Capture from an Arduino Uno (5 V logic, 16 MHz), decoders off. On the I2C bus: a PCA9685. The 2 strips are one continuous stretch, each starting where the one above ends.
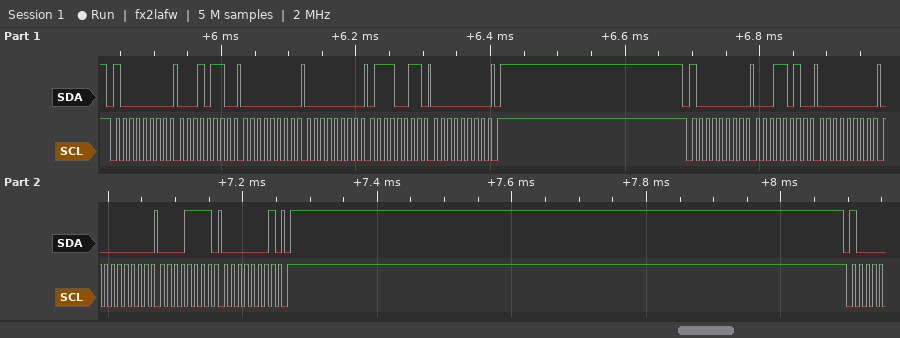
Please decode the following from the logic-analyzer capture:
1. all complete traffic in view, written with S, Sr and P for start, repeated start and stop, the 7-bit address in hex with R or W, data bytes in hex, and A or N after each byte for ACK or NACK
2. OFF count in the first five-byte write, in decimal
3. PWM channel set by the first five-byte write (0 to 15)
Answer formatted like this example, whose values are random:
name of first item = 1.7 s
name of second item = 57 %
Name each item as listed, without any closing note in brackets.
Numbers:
all complete traffic in view, written with S, Sr and P for start, repeated start and stop, the 7-bit address in hex with R or W, data bytes in hex, and A or N after each byte for ACK or NACK = S 40W A 16 A 00 A 00 A 73 A 00 A P S 40W A 1A A 00 A 00 A 0F A 01 A P
OFF count in the first five-byte write, in decimal = 115
PWM channel set by the first five-byte write = 4
